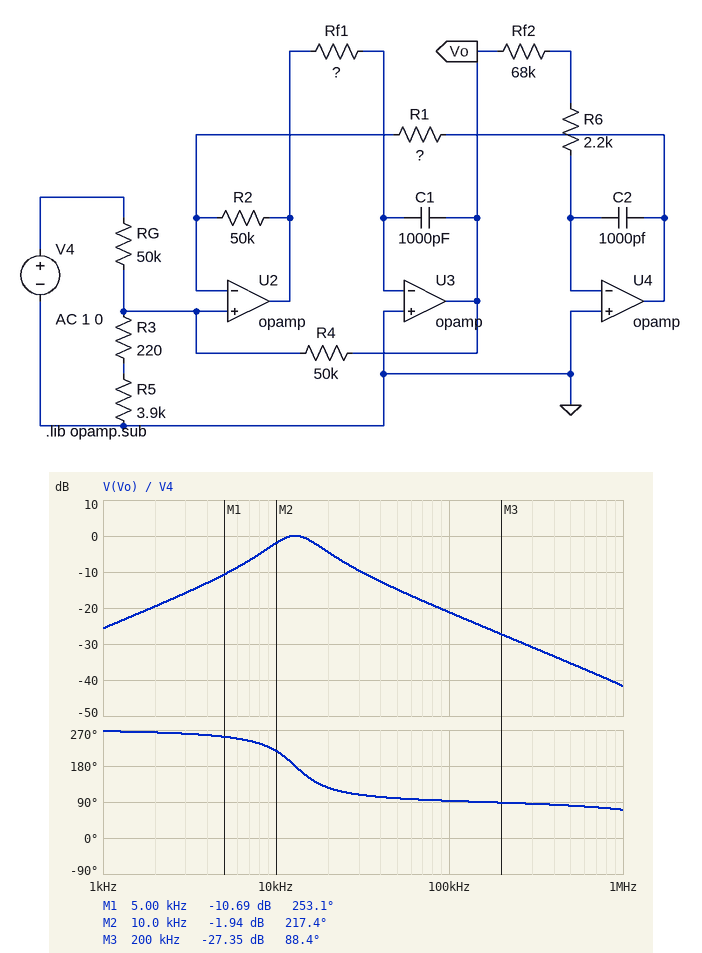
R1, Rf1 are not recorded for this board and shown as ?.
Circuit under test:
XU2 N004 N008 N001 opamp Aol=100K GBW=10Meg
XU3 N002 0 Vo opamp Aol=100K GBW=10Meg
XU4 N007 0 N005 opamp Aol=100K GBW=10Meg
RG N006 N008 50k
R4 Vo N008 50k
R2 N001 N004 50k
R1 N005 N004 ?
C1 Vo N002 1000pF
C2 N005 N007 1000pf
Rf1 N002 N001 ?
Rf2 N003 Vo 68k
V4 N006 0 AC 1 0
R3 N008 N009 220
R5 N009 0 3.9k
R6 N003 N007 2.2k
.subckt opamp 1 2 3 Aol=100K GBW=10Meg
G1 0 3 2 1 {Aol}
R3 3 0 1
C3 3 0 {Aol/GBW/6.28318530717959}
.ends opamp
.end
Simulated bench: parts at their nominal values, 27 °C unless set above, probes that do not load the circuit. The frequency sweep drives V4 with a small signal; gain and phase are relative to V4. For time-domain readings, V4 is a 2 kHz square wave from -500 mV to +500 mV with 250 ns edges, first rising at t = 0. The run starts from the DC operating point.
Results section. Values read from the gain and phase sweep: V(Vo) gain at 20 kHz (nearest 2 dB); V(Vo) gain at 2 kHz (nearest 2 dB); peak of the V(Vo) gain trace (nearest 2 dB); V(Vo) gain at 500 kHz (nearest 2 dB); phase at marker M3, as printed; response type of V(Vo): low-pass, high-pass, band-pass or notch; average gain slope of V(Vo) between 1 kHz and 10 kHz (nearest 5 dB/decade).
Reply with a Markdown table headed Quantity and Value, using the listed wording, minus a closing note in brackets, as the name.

| Quantity | Value |
|---|---|
| V(Vo) gain at 20 kHz | -4 dB |
| V(Vo) gain at 2 kHz | -20 dB |
| peak of the V(Vo) gain trace | 0 dB |
| V(Vo) gain at 500 kHz | -36 dB |
| phase at marker M3, as printed | 88.4 deg |
| response type of V(Vo): low-pass, high-pass, band-pass or notch | band-pass |
| average gain slope of V(Vo) between 1 kHz and 10 kHz | 25 dB/decade |
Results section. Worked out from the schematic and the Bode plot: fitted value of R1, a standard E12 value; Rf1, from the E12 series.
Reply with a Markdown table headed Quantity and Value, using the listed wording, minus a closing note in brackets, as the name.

| Quantity | Value |
|---|---|
| fitted value of R1, a standard E12 value | 33 kΩ |
| Rf1, from the E12 series | 3.3 kΩ |
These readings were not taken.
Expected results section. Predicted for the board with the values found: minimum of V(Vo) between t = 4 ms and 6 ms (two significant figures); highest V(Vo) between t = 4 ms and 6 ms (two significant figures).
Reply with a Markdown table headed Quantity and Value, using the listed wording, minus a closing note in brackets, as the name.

| Quantity | Value |
|---|---|
| minimum of V(Vo) between t = 4 ms and 6 ms | -430 mV |
| highest V(Vo) between t = 4 ms and 6 ms | 430 mV |
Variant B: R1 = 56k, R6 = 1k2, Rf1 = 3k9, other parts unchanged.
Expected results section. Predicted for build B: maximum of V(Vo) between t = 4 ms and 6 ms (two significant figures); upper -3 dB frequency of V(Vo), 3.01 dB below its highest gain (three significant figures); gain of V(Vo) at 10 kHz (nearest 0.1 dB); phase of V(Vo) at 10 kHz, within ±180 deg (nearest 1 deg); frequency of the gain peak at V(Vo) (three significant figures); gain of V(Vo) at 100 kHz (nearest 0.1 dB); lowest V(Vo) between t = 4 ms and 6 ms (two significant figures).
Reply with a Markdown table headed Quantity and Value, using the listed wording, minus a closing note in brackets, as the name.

| Quantity | Value |
|---|---|
| maximum of V(Vo) between t = 4 ms and 6 ms | 400 mV |
| upper -3 dB frequency of V(Vo), 3.01 dB below its highest gain | 12.2 kHz |
| gain of V(Vo) at 10 kHz | -0.3 dB |
| phase of V(Vo) at 10 kHz, within ±180 deg | 163 deg |
| frequency of the gain peak at V(Vo) | 9.14 kHz |
| gain of V(Vo) at 100 kHz | -25.2 dB |
| lowest V(Vo) between t = 4 ms and 6 ms | -400 mV |
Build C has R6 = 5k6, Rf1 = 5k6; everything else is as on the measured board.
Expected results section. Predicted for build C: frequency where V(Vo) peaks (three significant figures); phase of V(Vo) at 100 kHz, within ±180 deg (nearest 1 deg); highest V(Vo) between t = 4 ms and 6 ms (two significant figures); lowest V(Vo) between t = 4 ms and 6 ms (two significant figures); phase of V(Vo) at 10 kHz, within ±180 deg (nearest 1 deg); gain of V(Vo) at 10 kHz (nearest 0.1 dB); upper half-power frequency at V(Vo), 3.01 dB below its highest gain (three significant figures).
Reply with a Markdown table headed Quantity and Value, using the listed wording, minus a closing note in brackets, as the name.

| Quantity | Value |
|---|---|
| frequency where V(Vo) peaks | 9.64 kHz |
| phase of V(Vo) at 100 kHz, within ±180 deg | 91 deg |
| highest V(Vo) between t = 4 ms and 6 ms | 370 mV |
| lowest V(Vo) between t = 4 ms and 6 ms | -370 mV |
| phase of V(Vo) at 10 kHz, within ±180 deg | 172 deg |
| gain of V(Vo) at 10 kHz | 0 dB |
| upper half-power frequency at V(Vo), 3.01 dB below its highest gain | 12.5 kHz |
